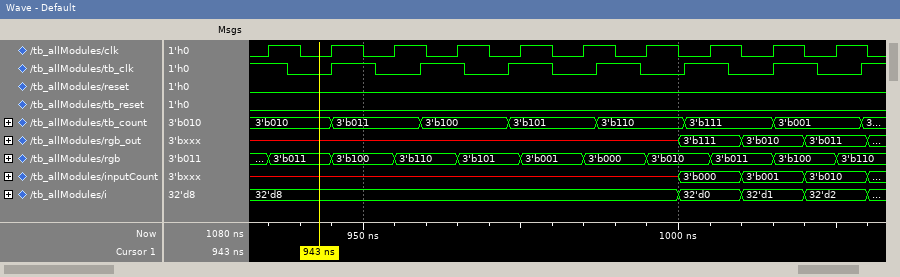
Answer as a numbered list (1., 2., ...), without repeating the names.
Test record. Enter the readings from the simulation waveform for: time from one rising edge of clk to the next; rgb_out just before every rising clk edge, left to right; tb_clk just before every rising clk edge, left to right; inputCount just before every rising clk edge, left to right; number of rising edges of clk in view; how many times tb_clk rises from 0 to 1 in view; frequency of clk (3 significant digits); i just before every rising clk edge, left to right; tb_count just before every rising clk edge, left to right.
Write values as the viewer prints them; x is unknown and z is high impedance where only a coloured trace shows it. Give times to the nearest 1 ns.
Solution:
1. 10 ns
2. x, x, x, x, x, x, x, 3'b111, 3'b010, 3'b011
3. 1 0 0 1 1 0 0 1 0 0
4. x, x, x, x, x, x, x, 3'b000, 3'b001, 3'b010
5. 10
6. 7
7. 100 MHz
8. 32'd8, 32'd8, 32'd8, 32'd8, 32'd8, 32'd8, 32'd8, 32'd0, 32'd1, 32'd2
9. 3'b010, 3'b010, 3'b011, 3'b100, 3'b101, 3'b101, 3'b110, 3'b111, 3'b111, 3'b001
